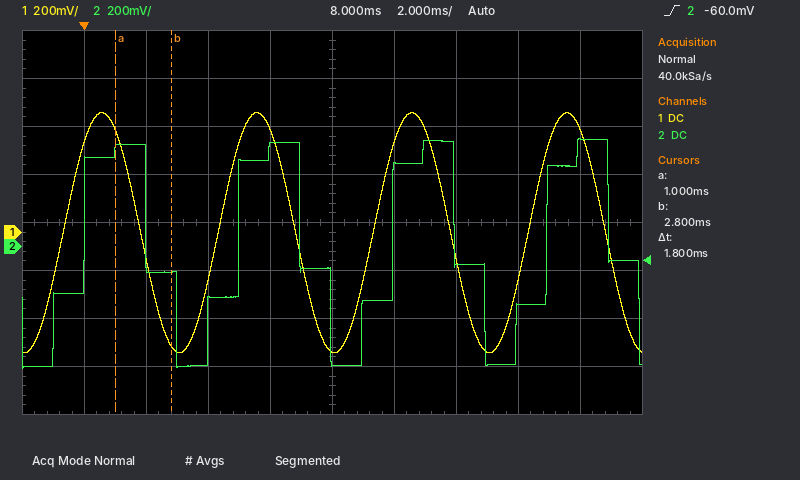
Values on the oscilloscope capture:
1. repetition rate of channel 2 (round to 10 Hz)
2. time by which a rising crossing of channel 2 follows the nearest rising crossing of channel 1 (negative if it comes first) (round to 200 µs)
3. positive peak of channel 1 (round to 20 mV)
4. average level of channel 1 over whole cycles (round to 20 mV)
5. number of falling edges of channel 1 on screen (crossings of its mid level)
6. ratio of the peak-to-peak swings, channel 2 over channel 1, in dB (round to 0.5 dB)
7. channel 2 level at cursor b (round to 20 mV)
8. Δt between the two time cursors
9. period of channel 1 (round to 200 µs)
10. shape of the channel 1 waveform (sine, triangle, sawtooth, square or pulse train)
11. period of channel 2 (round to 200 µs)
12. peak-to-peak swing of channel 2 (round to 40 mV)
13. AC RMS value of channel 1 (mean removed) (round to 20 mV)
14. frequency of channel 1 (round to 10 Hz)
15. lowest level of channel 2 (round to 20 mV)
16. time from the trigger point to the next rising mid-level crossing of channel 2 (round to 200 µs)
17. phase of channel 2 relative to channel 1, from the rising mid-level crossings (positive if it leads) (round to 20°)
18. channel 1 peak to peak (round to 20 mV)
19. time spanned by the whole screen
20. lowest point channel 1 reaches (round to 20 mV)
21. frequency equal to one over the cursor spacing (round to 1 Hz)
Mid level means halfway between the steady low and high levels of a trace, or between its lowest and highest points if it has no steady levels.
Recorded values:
200 Hz
+600 µs
500 mV
0 mV
4
-0.5 dB
-100 mV
1.8 ms
5.0 ms
sine
5.0 ms
960 mV
360 mV
200 Hz
-500 mV
5.0 ms
-40°
1.00 V
20 ms
-500 mV
556 Hz
